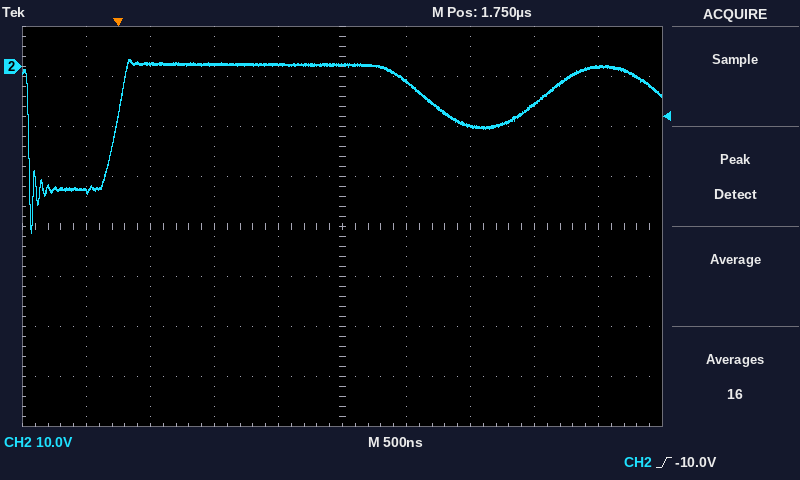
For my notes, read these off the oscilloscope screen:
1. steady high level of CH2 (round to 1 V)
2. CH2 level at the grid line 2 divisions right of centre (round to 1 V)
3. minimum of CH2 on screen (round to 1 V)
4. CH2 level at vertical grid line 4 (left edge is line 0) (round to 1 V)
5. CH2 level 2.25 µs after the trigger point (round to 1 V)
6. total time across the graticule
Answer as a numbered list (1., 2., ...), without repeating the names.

1. 0 V
2. -12 V
3. -33 V
4. 0 V
5. -3 V
6. 5 µs
